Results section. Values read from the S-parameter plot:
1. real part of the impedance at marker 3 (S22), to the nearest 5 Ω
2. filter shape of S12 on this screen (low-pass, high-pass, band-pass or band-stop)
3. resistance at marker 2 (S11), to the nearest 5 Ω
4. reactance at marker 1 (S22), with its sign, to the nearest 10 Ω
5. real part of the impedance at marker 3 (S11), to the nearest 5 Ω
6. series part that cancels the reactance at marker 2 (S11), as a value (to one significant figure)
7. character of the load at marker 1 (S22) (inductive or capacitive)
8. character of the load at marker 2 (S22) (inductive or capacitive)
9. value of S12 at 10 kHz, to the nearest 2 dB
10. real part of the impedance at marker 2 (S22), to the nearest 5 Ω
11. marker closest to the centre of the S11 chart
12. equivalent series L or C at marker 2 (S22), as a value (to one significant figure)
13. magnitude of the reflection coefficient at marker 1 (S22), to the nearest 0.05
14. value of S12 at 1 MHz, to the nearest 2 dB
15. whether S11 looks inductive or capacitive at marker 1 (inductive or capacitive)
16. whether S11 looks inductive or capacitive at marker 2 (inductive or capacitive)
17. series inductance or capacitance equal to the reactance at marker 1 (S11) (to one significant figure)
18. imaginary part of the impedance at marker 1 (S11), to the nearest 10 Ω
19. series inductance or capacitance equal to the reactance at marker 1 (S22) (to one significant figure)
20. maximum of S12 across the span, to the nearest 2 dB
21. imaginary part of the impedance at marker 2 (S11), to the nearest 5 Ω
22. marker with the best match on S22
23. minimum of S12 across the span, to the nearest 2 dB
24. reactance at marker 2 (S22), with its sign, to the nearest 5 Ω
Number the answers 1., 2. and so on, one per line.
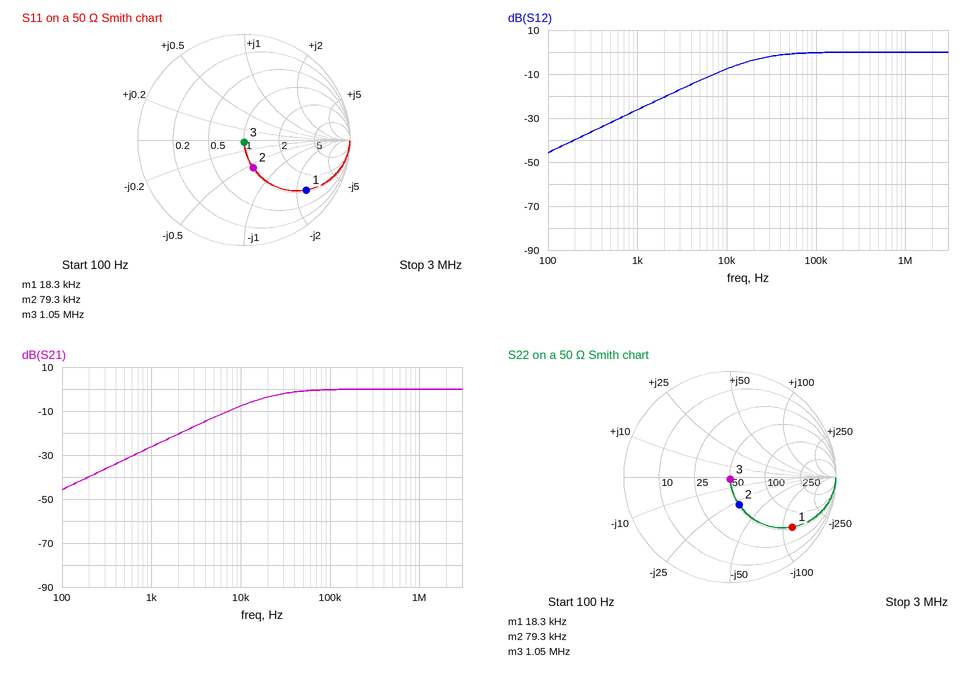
1. 50 Ω
2. high-pass
3. 50 Ω
4. -120 Ω
5. 50 Ω
6. 60 µH
7. capacitive
8. capacitive
9. -8 dB
10. 50 Ω
11. marker 3
12. 70 nF
13. 0.75
14. 0 dB
15. capacitive
16. capacitive
17. 70 nF
18. -120 Ω
19. 70 nF
20. 0 dB
21. -30 Ω
22. marker 3
23. -46 dB
24. -30 Ω
